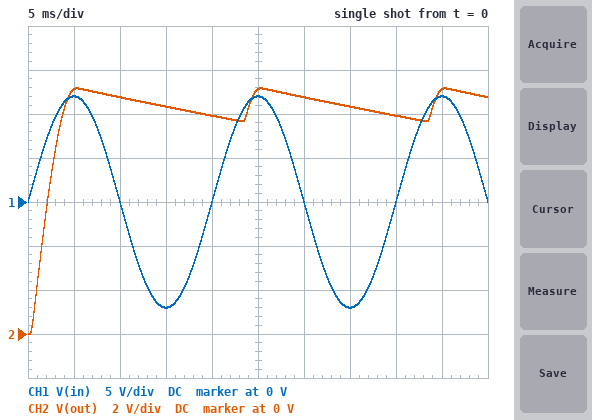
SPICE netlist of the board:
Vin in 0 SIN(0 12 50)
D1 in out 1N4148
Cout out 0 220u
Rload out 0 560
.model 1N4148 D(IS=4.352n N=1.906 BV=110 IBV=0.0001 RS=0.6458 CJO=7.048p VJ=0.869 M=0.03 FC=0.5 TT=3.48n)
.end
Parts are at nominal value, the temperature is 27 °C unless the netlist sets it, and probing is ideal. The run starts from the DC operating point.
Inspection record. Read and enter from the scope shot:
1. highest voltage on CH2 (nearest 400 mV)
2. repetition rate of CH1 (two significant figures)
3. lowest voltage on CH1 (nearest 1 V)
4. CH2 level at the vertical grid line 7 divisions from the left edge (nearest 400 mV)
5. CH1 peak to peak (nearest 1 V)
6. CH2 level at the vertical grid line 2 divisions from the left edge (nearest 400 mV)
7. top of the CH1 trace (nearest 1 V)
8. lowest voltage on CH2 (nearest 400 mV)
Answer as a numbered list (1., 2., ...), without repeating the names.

1. 11.2 V
2. 50 Hz
3. -12 V
4. 10.4 V
5. 24 V
6. 10.8 V
7. 12 V
8. 0 V
